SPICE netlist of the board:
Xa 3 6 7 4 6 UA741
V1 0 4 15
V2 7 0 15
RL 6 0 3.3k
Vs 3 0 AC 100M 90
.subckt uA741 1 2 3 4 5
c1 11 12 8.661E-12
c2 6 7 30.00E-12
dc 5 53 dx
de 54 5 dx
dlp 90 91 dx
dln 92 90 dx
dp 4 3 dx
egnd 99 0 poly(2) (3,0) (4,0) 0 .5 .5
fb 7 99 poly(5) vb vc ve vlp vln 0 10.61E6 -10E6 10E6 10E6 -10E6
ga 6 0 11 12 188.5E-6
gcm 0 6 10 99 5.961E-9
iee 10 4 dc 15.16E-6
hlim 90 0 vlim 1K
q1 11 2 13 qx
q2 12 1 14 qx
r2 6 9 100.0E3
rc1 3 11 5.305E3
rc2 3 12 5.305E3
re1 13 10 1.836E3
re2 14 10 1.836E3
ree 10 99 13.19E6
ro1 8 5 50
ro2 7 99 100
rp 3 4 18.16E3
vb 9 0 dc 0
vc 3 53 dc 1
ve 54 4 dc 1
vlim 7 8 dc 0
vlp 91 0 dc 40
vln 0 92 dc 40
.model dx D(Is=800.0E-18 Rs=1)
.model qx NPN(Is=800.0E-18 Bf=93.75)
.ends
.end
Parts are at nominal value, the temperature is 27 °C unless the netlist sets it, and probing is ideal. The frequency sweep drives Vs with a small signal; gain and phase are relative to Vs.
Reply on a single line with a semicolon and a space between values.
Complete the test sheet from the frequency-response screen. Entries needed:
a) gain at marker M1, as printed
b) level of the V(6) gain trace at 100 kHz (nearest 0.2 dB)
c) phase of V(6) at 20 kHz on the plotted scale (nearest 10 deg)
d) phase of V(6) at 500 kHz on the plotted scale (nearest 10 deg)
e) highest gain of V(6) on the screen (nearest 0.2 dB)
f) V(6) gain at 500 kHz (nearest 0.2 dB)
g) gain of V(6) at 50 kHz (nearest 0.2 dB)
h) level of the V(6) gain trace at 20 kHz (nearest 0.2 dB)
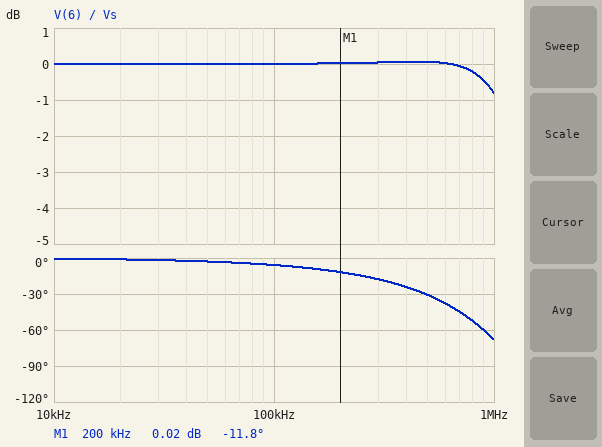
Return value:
0.02 dB; 0 dB; 0 deg; -30 deg; 0 dB; 0 dB; 0 dB; 0 dB
